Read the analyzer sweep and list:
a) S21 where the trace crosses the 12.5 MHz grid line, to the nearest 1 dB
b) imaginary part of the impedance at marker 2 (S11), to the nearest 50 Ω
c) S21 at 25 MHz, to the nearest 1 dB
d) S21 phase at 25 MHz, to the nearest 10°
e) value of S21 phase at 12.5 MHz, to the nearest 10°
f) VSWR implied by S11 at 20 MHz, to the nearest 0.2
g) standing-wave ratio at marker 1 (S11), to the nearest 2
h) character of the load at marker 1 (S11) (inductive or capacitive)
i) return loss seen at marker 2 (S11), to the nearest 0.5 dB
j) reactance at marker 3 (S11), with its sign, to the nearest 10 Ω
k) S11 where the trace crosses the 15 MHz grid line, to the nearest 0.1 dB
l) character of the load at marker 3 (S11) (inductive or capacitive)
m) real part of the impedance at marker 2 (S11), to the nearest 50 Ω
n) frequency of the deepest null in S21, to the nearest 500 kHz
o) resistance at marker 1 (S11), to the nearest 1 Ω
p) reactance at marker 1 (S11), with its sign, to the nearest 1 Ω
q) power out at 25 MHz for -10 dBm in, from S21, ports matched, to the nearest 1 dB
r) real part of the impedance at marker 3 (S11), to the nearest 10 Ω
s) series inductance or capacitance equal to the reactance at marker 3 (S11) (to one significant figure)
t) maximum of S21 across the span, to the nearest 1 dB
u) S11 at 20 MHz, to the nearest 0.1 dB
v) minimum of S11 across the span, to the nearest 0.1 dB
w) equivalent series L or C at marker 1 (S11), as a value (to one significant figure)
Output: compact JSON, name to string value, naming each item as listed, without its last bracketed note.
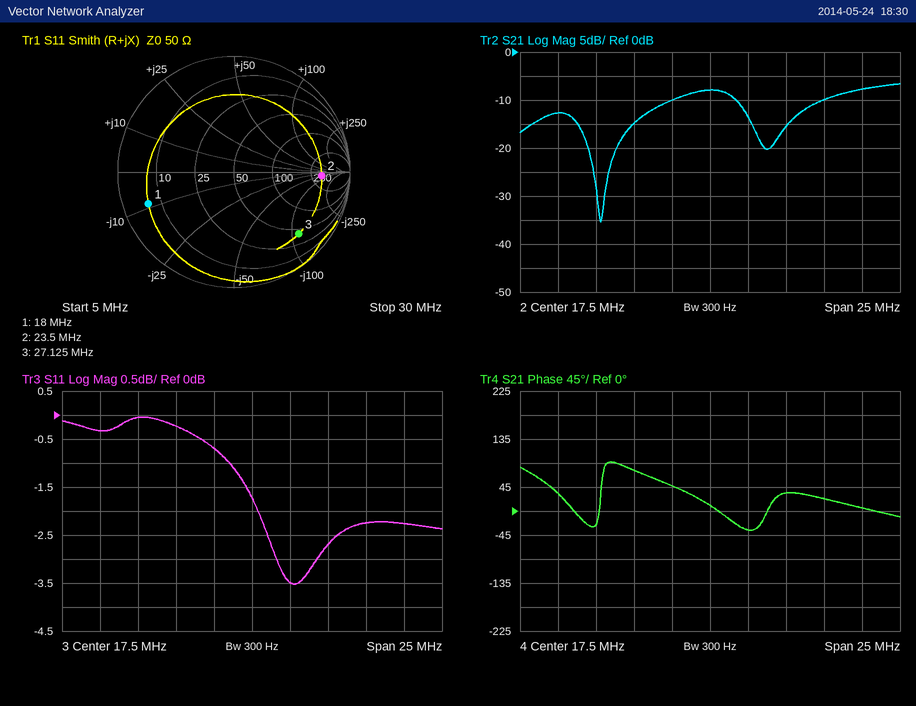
{"S21 where the trace crosses the 12.5 MHz grid line, to the nearest 1 dB": "-15 dB", "imaginary part of the impedance at marker 2 (S11), to the nearest 50 Ω": "-50 Ω", "S21 at 25 MHz, to the nearest 1 dB": "-10 dB", "S21 phase at 25 MHz, to the nearest 10°": "20°", "value of S21 phase at 12.5 MHz, to the nearest 10°": "80°", "VSWR implied by S11 at 20 MHz, to the nearest 0.2": "5.0", "standing-wave ratio at marker 1 (S11), to the nearest 2": "8", "character of the load at marker 1 (S11)": "capacitive", "return loss seen at marker 2 (S11), to the nearest 0.5 dB": "2.5 dB", "reactance at marker 3 (S11), with its sign, to the nearest 10 Ω": "-110 Ω", "S11 where the trace crosses the 15 MHz grid line, to the nearest 0.1 dB": "-0.7 dB", "character of the load at marker 3 (S11)": "capacitive", "real part of the impedance at marker 2 (S11), to the nearest 50 Ω": "350 Ω", "frequency of the deepest null in S21, to the nearest 500 kHz": "10.5 MHz", "resistance at marker 1 (S11), to the nearest 1 Ω": "6 Ω", "reactance at marker 1 (S11), with its sign, to the nearest 1 Ω": "-9 Ω", "power out at 25 MHz for -10 dBm in, from S21, ports matched, to the nearest 1 dB": "-20 dBm", "real part of the impedance at marker 3 (S11), to the nearest 10 Ω": "40 Ω", "series inductance or capacitance equal to the reactance at marker 3 (S11)": "50 pF", "maximum of S21 across the span, to the nearest 1 dB": "-7 dB", "S11 at 20 MHz, to the nearest 0.1 dB": "-3.5 dB", "minimum of S11 across the span, to the nearest 0.1 dB": "-3.5 dB", "equivalent series L or C at marker 1 (S11), as a value": "1.0 nF"}
